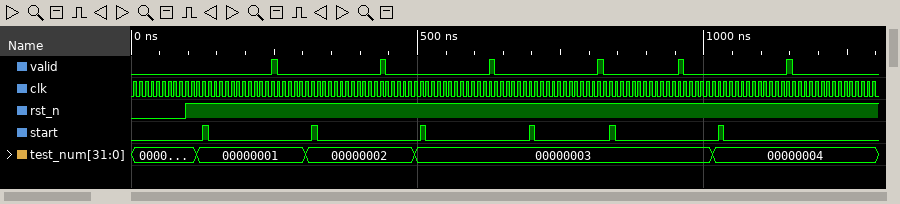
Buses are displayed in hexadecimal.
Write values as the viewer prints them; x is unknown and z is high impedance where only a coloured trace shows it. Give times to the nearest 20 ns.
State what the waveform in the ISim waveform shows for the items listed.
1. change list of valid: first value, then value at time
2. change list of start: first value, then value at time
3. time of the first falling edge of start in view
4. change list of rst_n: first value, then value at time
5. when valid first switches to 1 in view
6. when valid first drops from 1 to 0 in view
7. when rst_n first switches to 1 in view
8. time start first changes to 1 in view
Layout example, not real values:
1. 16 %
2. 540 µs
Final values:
1. 0, 1 at 240 ns, 0 at 260 ns, 1 at 440 ns, 0 at 440 ns, 1 at 620 ns, 0 at 640 ns, 1 at 820 ns, 0 at 820 ns, 1 at 960 ns, 0 at 960 ns, 1 at 1140 ns, 0 at 1160 ns
2. 0, 1 at 120 ns, 0 at 140 ns, 1 at 320 ns, 0 at 320 ns, 1 at 500 ns, 0 at 520 ns, 1 at 700 ns, 0 at 700 ns, 1 at 840 ns, 0 at 840 ns, 1 at 1020 ns, 0 at 1040 ns
3. 140 ns
4. 0, 1 at 100 ns
5. 240 ns
6. 260 ns
7. 100 ns
8. 120 ns
